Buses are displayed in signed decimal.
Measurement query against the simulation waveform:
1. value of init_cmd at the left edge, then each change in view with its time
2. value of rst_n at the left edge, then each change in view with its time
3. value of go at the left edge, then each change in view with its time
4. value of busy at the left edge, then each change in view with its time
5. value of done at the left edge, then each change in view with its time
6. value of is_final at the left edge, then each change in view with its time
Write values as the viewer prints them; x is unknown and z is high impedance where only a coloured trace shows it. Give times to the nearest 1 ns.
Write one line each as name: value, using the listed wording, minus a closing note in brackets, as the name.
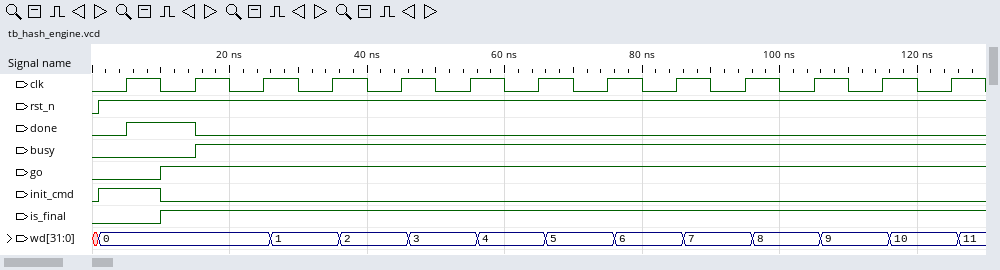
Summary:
value of init_cmd at the left edge, then each change in view with its time: 0, 1 at 1 ns, 0 at 10 ns
value of rst_n at the left edge, then each change in view with its time: 0, 1 at 1 ns
value of go at the left edge, then each change in view with its time: 0, 1 at 10 ns
value of busy at the left edge, then each change in view with its time: 0, 1 at 15 ns
value of done at the left edge, then each change in view with its time: 0, 1 at 5 ns, 0 at 15 ns
value of is_final at the left edge, then each change in view with its time: 0, 1 at 10 ns
